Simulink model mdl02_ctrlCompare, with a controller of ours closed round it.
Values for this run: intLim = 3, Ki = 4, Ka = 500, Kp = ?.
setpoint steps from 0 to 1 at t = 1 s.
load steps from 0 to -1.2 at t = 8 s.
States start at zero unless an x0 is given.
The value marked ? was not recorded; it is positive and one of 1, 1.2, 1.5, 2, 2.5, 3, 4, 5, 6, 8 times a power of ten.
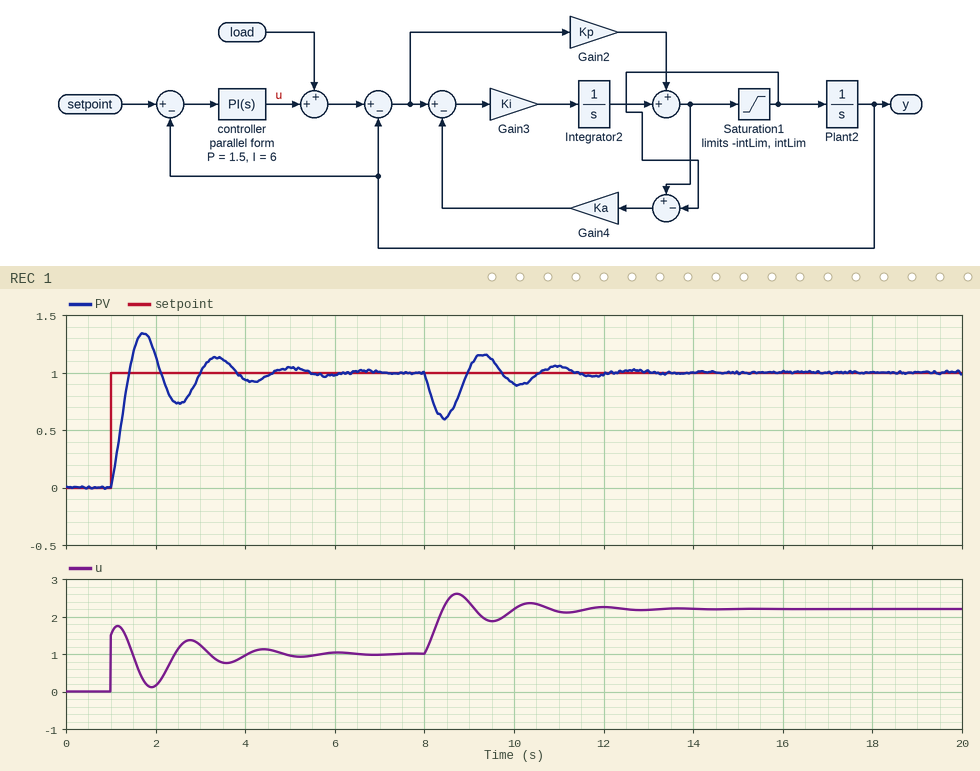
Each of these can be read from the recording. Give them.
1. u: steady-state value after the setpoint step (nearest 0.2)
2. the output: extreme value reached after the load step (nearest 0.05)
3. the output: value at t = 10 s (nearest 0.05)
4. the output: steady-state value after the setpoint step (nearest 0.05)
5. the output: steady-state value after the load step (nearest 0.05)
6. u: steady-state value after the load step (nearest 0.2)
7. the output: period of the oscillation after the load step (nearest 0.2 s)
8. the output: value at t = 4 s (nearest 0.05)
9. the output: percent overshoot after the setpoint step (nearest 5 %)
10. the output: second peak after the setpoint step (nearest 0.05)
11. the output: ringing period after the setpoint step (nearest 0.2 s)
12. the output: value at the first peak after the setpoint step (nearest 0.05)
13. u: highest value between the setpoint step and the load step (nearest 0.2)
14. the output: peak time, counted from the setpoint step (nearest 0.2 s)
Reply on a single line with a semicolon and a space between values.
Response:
1.0; 0.60; 0.90; 1.00; 1.00; 2.2; 1.6 s; 0.95; 35 %; 1.15; 1.6 s; 1.35; 1.8; 0.8 s
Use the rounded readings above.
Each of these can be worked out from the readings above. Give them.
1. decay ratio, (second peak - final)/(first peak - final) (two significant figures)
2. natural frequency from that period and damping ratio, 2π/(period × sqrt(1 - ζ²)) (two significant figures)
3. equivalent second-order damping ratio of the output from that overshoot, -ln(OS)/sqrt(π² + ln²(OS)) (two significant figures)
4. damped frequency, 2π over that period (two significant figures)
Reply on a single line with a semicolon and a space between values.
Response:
0.43; 4.1 rad/s; 0.32; 3.9 rad/s
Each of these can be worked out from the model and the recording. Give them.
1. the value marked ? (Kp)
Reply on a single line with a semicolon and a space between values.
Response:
1.2
